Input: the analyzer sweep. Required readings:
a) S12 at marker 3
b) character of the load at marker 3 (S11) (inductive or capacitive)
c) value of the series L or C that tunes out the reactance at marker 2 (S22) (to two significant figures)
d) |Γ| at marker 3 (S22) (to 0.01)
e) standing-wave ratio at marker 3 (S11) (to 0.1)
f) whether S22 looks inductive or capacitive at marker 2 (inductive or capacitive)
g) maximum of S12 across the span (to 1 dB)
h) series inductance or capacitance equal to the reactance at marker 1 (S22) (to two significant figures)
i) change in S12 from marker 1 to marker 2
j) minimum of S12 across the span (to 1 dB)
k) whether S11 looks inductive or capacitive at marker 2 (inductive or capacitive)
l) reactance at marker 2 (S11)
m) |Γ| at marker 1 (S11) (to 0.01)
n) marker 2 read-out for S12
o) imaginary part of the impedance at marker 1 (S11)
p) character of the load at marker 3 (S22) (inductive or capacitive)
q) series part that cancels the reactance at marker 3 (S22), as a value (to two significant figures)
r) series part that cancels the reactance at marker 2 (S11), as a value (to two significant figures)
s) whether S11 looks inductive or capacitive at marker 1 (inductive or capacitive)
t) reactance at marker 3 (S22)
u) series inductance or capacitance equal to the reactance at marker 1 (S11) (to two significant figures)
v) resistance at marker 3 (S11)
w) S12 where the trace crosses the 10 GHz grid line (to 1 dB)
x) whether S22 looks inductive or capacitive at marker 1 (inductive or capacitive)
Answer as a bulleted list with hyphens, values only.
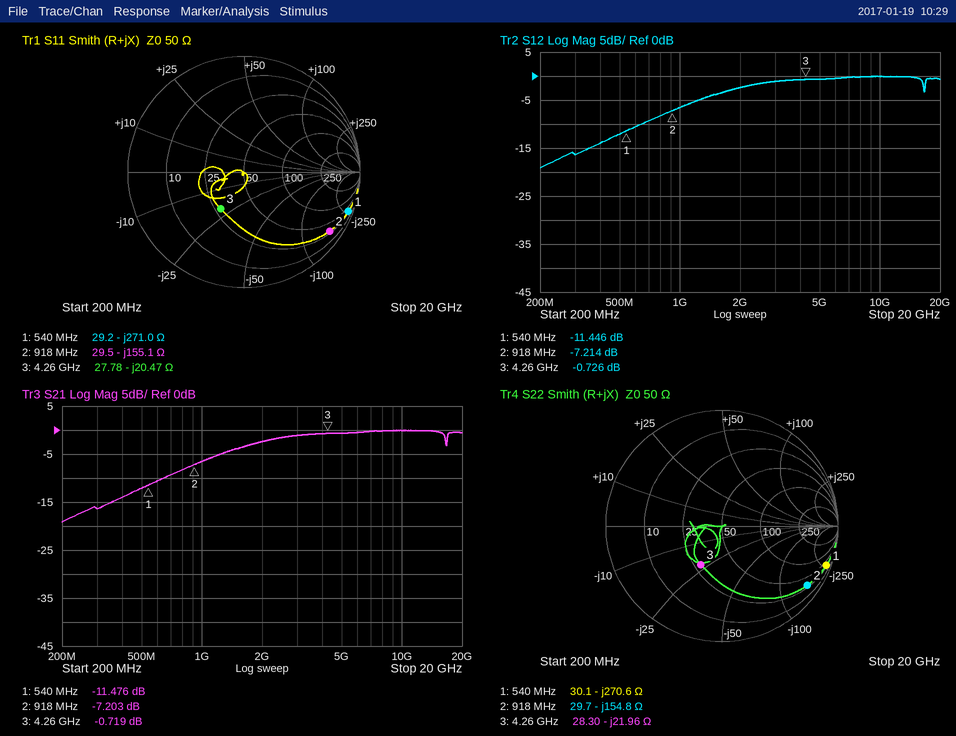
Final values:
- -0.726 dB
- capacitive
- 27 nH
- 0.38
- 2.2
- capacitive
- 0 dB
- 1.1 pF
- 4.232 dB
- -19 dB
- capacitive
- -155.1 Ω
- 0.96
- -7.214 dB
- -271.0 Ω
- capacitive
- 820 pH
- 27 nH
- capacitive
- -21.96 Ω
- 1.1 pF
- 27.78 Ω
- 0 dB
- capacitive
